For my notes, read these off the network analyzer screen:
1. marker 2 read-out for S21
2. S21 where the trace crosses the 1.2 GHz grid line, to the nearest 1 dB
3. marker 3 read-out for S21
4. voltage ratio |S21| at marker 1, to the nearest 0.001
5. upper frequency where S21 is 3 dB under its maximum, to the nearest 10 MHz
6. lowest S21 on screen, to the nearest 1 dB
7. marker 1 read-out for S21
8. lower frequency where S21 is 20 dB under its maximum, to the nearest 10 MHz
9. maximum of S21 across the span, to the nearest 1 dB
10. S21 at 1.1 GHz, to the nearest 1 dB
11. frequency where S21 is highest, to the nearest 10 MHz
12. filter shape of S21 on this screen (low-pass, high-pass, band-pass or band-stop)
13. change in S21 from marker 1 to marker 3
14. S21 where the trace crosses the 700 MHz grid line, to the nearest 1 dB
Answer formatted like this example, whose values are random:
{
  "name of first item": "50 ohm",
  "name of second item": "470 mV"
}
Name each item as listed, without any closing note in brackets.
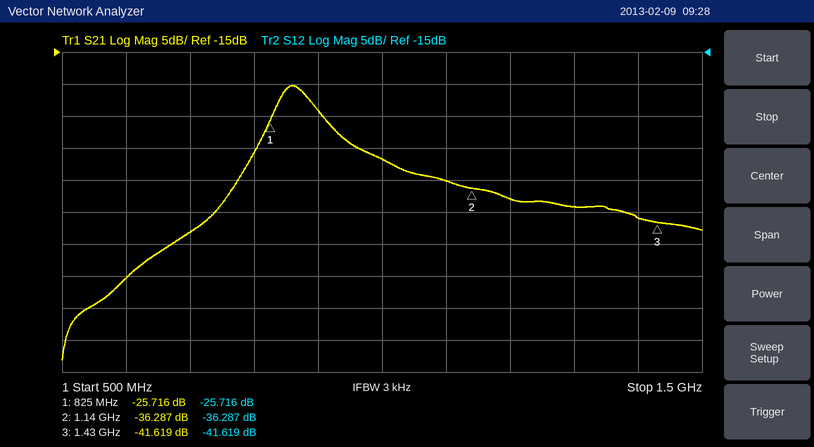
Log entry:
{
  "marker 2 read-out for S21": "-36.287 dB",
  "S21 where the trace crosses the 1.2 GHz grid line, to the nearest 1 dB": "-38 dB",
  "marker 3 read-out for S21": "-41.619 dB",
  "voltage ratio |S21| at marker 1, to the nearest 0.001": "0.052",
  "upper frequency where S21 is 3 dB under its maximum, to the nearest 10 MHz": "890 MHz",
  "lowest S21 on screen, to the nearest 1 dB": "-63 dB",
  "marker 1 read-out for S21": "-25.716 dB",
  "lower frequency where S21 is 20 dB under its maximum, to the nearest 10 MHz": "740 MHz",
  "maximum of S21 across the span, to the nearest 1 dB": "-20 dB",
  "S21 at 1.1 GHz, to the nearest 1 dB": "-35 dB",
  "frequency where S21 is highest, to the nearest 10 MHz": "860 MHz",
  "filter shape of S21 on this screen": "band-pass",
  "change in S21 from marker 1 to marker 3": "-15.903 dB",
  "S21 where the trace crosses the 700 MHz grid line, to the nearest 1 dB": "-43 dB"
}
